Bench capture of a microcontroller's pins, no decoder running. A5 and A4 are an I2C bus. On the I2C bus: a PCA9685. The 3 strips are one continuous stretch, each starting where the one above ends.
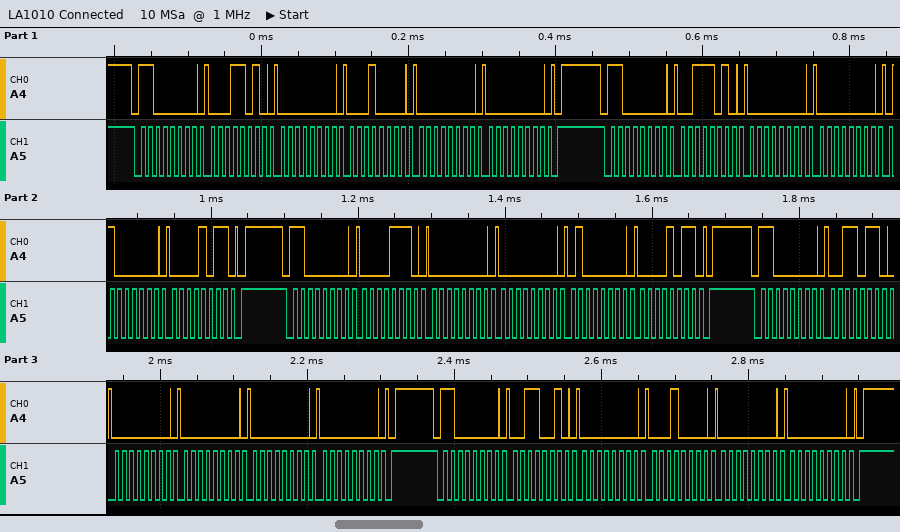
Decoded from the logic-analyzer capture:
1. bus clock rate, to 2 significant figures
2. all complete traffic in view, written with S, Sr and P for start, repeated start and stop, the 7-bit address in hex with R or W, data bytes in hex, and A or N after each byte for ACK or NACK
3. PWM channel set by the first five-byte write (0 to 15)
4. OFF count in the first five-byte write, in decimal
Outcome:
100 kHz
S 60W A 1A A 00 A 10 A 00 A 00 A P S 60W A 3A A 00 A 00 A 40 A 0B A P S 60W A 0E A 00 A 00 A 40 A 0B A P S 60W A 36 A 00 A 00 A 00 A 00 A P S 60W A 32 A 00 A 10 A 00 A 00 A P
5
0
